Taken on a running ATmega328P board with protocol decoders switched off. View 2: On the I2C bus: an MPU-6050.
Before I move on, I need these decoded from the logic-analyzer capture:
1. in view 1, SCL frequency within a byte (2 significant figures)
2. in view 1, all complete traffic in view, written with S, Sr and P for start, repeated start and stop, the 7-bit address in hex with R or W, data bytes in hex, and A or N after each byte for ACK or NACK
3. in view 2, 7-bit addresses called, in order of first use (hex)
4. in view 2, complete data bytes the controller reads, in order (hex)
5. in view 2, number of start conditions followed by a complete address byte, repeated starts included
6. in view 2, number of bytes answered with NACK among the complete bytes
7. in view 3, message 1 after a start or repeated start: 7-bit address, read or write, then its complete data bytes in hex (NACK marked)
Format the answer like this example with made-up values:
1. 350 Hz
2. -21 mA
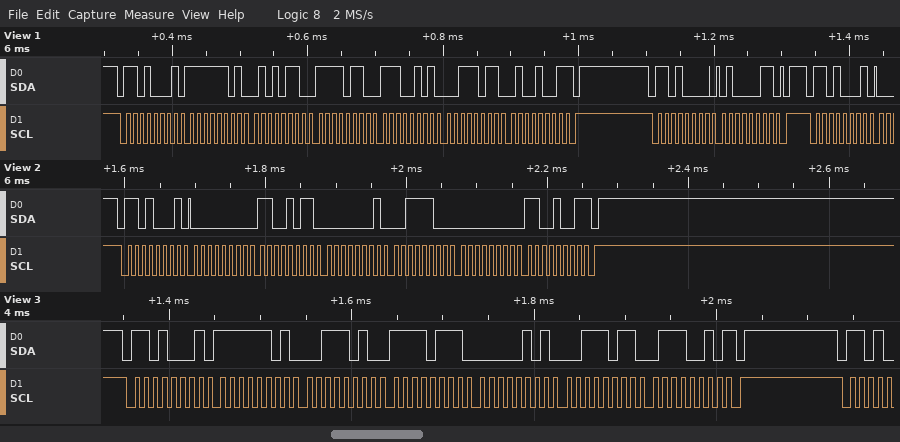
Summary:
1. 100 kHz
2. S 68R A FD A 56 A F6 A E5 A 3B A 49 N P S 68W A 43 A P S 68R A
3. 0x68
4. 00 CB 01 3C 00 C9
5. 1
6. 1
7. 0x68 read: FD 3A F7 05 3B 72 NACK
